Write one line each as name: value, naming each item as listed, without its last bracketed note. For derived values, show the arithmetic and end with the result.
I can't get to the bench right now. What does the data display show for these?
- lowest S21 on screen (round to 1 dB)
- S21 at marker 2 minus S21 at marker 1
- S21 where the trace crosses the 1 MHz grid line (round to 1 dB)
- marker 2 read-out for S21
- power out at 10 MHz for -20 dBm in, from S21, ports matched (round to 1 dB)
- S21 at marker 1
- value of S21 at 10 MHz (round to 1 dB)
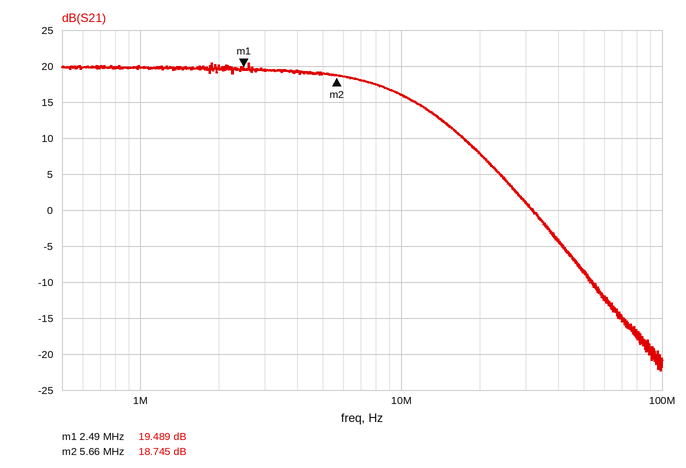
lowest S21 on screen: -22 dB
S21 at marker 2 minus S21 at marker 1: 18.745 − (19.489) = -0.744 dB
S21 where the trace crosses the 1 MHz grid line: 20 dB
marker 2 read-out for S21: 18.745 dB
power out at 10 MHz for -20 dBm in, from S21, ports matched: -20 dBm + (16 dB) = -4 dBm
S21 at marker 1: 19.489 dB
value of S21 at 10 MHz: 16 dB
